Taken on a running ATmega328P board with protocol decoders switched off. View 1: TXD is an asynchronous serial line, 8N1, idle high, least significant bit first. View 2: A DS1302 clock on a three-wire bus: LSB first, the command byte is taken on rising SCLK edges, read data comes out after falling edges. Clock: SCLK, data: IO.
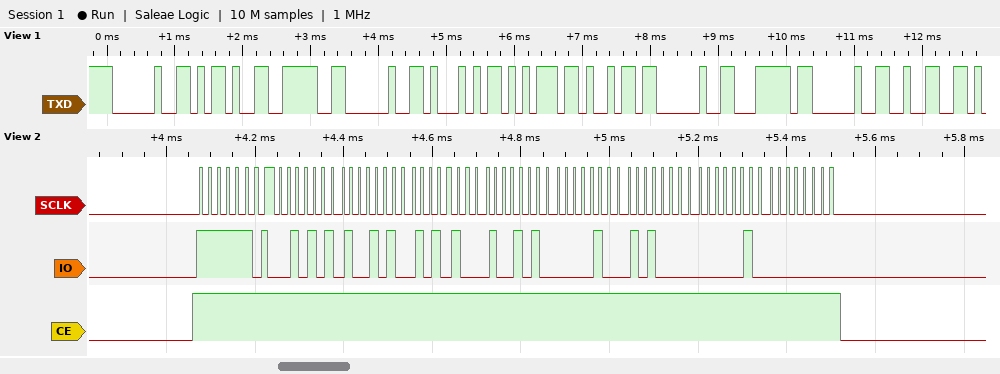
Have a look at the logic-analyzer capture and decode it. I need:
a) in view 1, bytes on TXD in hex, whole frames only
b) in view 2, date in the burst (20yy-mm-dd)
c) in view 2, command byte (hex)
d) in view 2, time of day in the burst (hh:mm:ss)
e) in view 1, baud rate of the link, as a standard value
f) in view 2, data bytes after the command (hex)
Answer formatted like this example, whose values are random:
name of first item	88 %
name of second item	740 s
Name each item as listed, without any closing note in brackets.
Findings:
in view 1, bytes on TXD in hex, whole frames only	20 2D 3E 20 51 75 69 20 7C 20 32
in view 2, date in the burst	2020-10-29
in view 2, command byte	0xBF
in view 2, time of day in the burst	15:29:54
in view 1, baud rate of the link, as a standard value	9600 baud
in view 2, data bytes after the command	54 29 15 29 10 05 20 00
